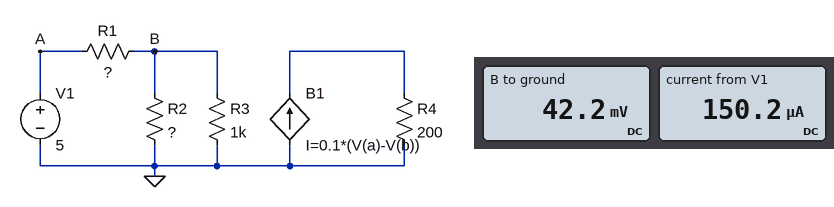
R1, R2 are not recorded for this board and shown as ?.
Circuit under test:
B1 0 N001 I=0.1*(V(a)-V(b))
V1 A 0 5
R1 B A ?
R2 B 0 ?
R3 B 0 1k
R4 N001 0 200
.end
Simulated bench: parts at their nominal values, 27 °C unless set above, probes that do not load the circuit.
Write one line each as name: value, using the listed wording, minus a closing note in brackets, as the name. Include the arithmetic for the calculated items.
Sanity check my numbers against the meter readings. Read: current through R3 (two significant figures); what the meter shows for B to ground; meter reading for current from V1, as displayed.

current through R3: (42.2 mV) / 1 kΩ = 42 µA
what the meter shows for B to ground: 42.2 mV
meter reading for current from V1, as displayed: 150.2 µA
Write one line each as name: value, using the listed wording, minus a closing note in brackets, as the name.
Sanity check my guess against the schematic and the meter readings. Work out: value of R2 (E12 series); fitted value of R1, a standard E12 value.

value of R2: 390 Ω
fitted value of R1, a standard E12 value: 33 kΩ
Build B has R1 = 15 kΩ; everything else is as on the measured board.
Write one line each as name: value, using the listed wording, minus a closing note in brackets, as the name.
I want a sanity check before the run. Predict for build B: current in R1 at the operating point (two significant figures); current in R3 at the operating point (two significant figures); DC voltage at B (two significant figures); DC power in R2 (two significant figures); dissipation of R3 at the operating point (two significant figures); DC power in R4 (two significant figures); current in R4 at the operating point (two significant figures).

current in R1 at the operating point: 330 µA
current in R3 at the operating point: 92 µA
DC voltage at B: 92 mV
DC power in R2: 22 µW
dissipation of R3 at the operating point: 8.4 µW
DC power in R4: 48 W
current in R4 at the operating point: 490 mA
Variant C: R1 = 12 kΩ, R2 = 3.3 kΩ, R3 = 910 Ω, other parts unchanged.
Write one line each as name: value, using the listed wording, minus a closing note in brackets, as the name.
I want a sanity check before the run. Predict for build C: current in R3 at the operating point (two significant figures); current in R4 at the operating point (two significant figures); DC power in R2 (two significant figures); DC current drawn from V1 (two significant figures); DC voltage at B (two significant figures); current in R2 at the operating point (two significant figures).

current in R3 at the operating point: 310 µA
current in R4 at the operating point: 470 mA
DC power in R2: 24 µW
DC current drawn from V1: 390 µA
DC voltage at B: 280 mV
current in R2 at the operating point: 85 µA
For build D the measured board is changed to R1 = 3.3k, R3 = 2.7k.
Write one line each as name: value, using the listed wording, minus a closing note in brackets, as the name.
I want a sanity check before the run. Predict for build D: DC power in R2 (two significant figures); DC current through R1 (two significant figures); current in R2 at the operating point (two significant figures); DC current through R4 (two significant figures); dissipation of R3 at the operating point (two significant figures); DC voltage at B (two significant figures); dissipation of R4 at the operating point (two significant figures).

DC power in R2: 560 µW
DC current through R1: 1.4 mA
current in R2 at the operating point: 1.2 mA
DC current through R4: 450 mA
dissipation of R3 at the operating point: 81 µW
DC voltage at B: 470 mV
dissipation of R4 at the operating point: 41 W
